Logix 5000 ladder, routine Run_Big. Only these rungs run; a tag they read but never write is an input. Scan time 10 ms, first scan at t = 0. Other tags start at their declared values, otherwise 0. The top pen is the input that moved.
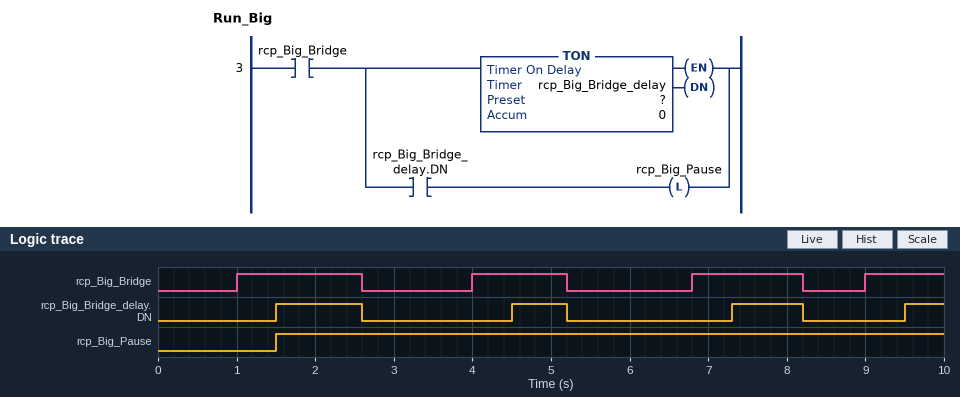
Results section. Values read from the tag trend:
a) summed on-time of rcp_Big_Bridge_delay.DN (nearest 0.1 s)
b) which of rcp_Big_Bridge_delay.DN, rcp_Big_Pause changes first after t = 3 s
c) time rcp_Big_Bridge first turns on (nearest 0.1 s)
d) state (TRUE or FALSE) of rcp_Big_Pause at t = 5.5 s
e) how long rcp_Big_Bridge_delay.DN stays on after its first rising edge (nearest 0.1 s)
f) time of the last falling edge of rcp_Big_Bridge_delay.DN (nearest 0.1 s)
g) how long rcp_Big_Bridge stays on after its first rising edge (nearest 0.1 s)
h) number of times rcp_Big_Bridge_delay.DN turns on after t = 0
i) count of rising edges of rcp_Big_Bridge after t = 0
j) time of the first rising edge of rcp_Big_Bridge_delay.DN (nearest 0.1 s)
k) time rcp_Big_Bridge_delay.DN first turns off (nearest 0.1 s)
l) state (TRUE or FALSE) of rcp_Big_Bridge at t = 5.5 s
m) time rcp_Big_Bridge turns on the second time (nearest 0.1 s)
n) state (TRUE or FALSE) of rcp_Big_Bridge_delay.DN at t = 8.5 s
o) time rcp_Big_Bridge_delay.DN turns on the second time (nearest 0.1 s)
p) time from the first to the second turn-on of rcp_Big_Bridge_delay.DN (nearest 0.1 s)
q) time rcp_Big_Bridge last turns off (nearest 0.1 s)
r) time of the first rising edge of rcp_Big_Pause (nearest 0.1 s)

3.2 s
rcp_Big_Bridge_delay.DN
1.0 s
TRUE
1.1 s
8.2 s
1.6 s
4
4
1.5 s
2.6 s
FALSE
4.0 s
FALSE
4.5 s
3.0 s
8.2 s
1.5 s
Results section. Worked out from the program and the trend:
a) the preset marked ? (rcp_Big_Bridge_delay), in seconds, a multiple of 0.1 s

0.5 s
